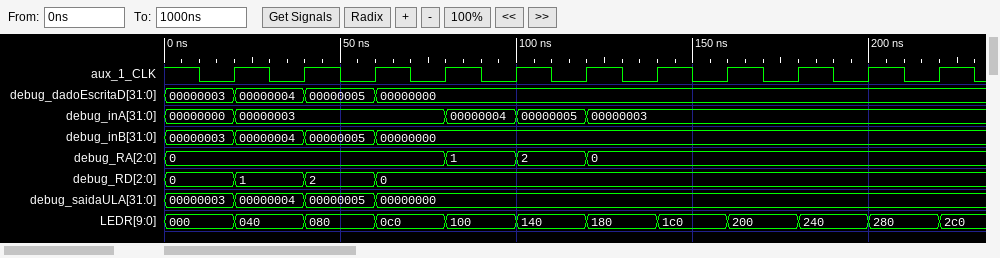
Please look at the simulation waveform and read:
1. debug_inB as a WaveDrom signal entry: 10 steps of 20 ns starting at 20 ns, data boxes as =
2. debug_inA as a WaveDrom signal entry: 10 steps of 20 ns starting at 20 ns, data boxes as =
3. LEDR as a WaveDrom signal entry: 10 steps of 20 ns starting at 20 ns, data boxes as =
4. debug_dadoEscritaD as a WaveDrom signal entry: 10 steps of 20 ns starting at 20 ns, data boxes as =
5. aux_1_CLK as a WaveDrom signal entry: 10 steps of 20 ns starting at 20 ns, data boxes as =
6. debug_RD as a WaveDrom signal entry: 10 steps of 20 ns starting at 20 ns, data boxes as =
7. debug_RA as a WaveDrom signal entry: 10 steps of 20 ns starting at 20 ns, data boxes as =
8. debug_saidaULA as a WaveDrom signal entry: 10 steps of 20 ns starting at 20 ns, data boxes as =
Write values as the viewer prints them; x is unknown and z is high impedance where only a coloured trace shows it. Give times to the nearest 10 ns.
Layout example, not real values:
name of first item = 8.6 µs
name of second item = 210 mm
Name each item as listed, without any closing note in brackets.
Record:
debug_inB as a WaveDrom signal entry: 10 steps of 20 ns starting at 20 ns, data boxes as = = {name: 'debug_inB', wave: '===.......', data: '00000004 00000005 00000000'}
debug_inA as a WaveDrom signal entry: 10 steps of 20 ns starting at 20 ns, data boxes as = = {name: 'debug_inA', wave: '=..===....', data: '00000003 00000004 00000005 00000003'}
LEDR as a WaveDrom signal entry: 10 steps of 20 ns starting at 20 ns, data boxes as = = {name: 'LEDR', wave: '==========', data: '040 080 0c0 100 140 180 1c0 200 240 280'}
debug_dadoEscritaD as a WaveDrom signal entry: 10 steps of 20 ns starting at 20 ns, data boxes as = = {name: 'debug_dadoEscritaD', wave: '===.......', data: '00000004 00000005 00000000'}
aux_1_CLK as a WaveDrom signal entry: 10 steps of 20 ns starting at 20 ns, data boxes as = = {name: 'aux_1_CLK', wave: 'p.........'}
debug_RD as a WaveDrom signal entry: 10 steps of 20 ns starting at 20 ns, data boxes as = = {name: 'debug_RD', wave: '===.......', data: '1 2 0'}
debug_RA as a WaveDrom signal entry: 10 steps of 20 ns starting at 20 ns, data boxes as = = {name: 'debug_RA', wave: '=..===....', data: '0 1 2 0'}
debug_saidaULA as a WaveDrom signal entry: 10 steps of 20 ns starting at 20 ns, data boxes as = = {name: 'debug_saidaULA', wave: '===.......', data: '00000004 00000005 00000000'}
